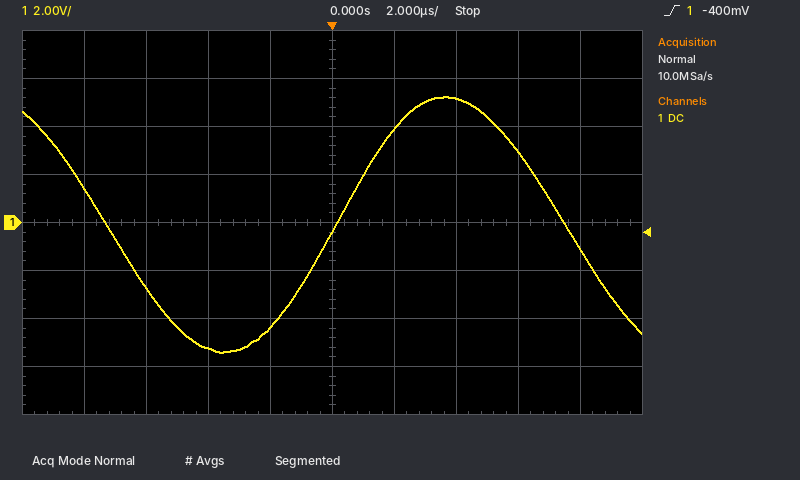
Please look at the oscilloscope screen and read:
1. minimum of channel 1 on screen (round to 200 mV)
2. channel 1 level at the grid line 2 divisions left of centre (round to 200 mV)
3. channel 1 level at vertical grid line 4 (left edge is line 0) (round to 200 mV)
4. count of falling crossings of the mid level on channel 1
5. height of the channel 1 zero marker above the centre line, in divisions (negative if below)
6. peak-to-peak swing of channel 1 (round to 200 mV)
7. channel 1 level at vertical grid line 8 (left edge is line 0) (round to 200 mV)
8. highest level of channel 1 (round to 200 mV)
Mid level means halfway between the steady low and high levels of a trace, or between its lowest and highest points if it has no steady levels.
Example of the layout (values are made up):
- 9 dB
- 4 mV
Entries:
- -5.4 V
- -5.2 V
- -4.4 V
- 2
- 0.0 div
- 10.6 V
- 3.0 V
- 5.2 V
